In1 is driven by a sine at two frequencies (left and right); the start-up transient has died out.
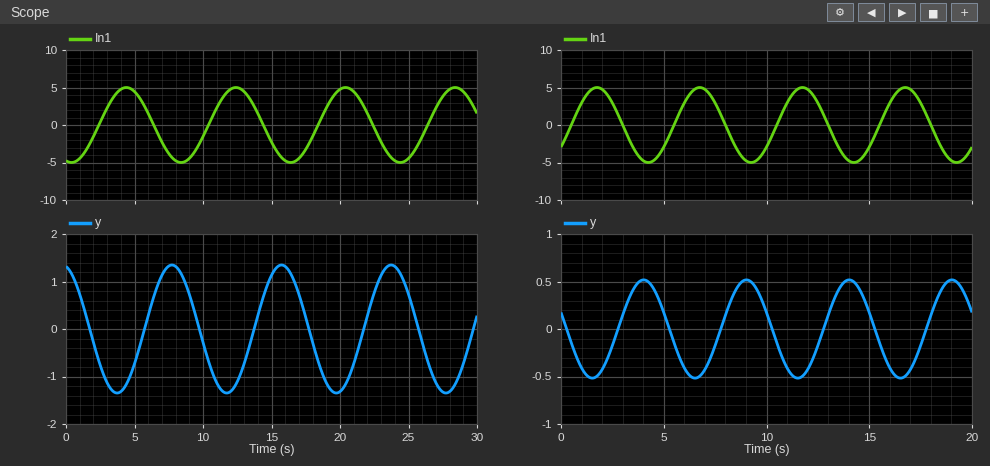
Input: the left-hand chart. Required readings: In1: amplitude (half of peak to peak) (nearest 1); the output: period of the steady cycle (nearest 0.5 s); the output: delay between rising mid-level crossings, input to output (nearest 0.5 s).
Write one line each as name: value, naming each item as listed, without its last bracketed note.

In1: amplitude (half of peak to peak): 5
the output: period of the steady cycle: 8.0 s
the output: delay between rising mid-level crossings, input to output: 3.5 s
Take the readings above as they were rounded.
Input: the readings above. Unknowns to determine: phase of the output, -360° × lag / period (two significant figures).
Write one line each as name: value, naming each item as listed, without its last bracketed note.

phase of the output, -360° × lag / period: -160°
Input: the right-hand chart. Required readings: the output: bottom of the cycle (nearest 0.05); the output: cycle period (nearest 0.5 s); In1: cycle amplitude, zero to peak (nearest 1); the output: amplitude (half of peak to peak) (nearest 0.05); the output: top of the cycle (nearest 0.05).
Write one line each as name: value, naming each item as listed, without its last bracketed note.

the output: bottom of the cycle: -0.50
the output: cycle period: 5.0 s
In1: cycle amplitude, zero to peak: 5
the output: amplitude (half of peak to peak): 0.50
the output: top of the cycle: 0.50
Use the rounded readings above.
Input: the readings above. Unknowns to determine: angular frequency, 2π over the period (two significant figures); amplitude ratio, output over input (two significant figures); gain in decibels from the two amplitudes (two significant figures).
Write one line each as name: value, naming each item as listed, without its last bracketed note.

angular frequency, 2π over the period: 1.3 rad/s
amplitude ratio, output over input: 0.10
gain in decibels from the two amplitudes: -20 dB
